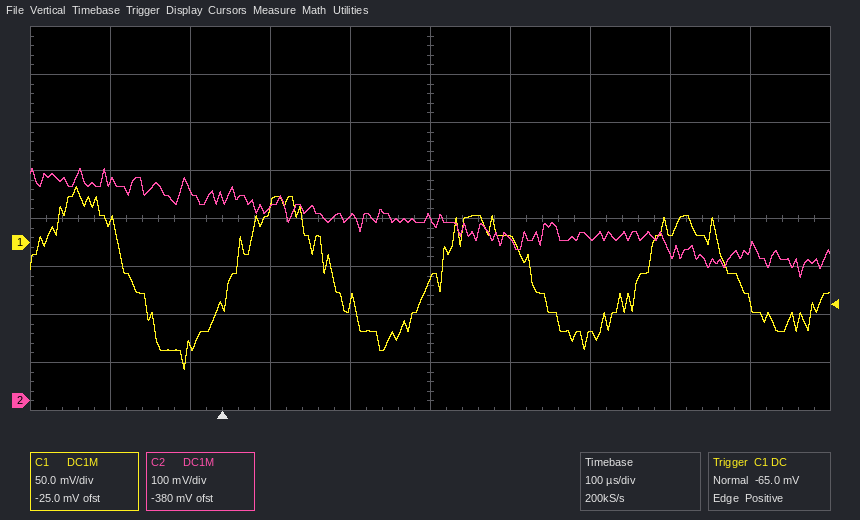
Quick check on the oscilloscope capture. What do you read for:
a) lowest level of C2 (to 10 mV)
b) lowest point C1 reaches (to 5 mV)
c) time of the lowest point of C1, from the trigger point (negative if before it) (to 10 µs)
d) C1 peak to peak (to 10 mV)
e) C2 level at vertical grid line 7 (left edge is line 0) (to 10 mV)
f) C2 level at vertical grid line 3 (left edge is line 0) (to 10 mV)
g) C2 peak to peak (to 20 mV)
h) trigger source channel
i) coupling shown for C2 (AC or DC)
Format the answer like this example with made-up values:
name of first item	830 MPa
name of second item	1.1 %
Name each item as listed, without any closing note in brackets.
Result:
lowest level of C2	260 mV
lowest point C1 reaches	-130 mV
time of the lowest point of C1, from the trigger point (negative if before it)	-50 µs
C1 peak to peak	190 mV
C2 level at vertical grid line 7 (left edge is line 0)	340 mV
C2 level at vertical grid line 3 (left edge is line 0)	400 mV
C2 peak to peak	220 mV
trigger source channel	C1
coupling shown for C2	DC
